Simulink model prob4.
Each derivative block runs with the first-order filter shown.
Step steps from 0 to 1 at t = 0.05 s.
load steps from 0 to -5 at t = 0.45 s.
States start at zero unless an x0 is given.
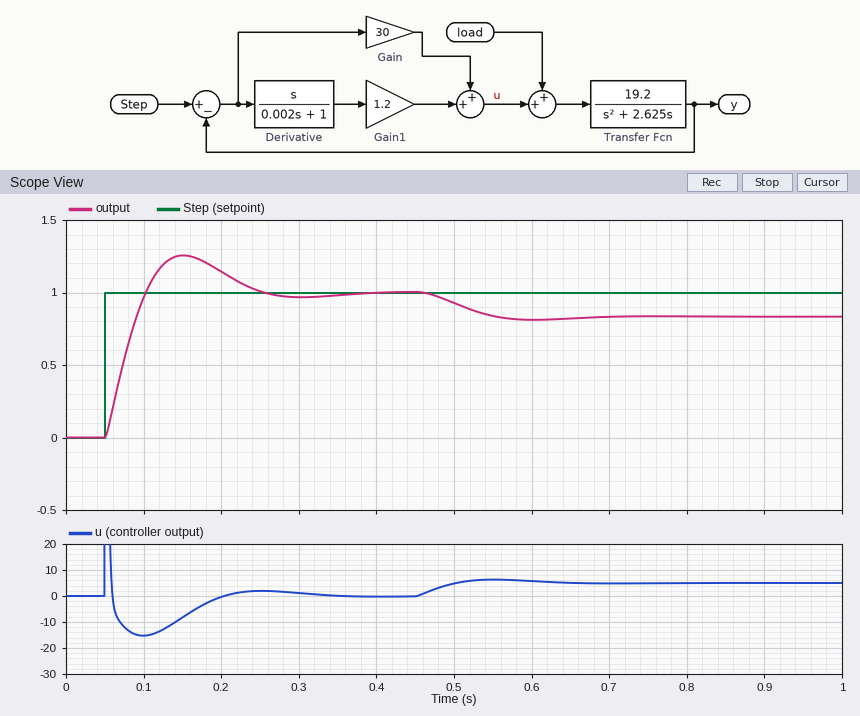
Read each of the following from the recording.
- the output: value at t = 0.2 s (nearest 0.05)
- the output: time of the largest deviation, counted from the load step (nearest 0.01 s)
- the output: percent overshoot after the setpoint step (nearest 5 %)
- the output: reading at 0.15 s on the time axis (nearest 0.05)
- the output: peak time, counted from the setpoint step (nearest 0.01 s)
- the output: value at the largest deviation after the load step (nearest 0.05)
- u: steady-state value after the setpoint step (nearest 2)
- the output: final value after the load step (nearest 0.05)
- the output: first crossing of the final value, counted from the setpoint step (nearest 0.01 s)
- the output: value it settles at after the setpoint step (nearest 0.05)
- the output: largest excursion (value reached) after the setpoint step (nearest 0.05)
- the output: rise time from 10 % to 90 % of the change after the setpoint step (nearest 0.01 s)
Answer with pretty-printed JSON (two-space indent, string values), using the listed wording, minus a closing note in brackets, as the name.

{
  "the output: value at t = 0.2 s": "1.15",
  "the output: time of the largest deviation, counted from the load step": "0.15 s",
  "the output: percent overshoot after the setpoint step": "25 %",
  "the output: reading at 0.15 s on the time axis": "1.25",
  "the output: peak time, counted from the setpoint step": "0.10 s",
  "the output: value at the largest deviation after the load step": "0.80",
  "u: steady-state value after the setpoint step": "0",
  "the output: final value after the load step": "0.85",
  "the output: first crossing of the final value, counted from the setpoint step": "0.05 s",
  "the output: value it settles at after the setpoint step": "1.00",
  "the output: largest excursion (value reached) after the setpoint step": "1.25",
  "the output: rise time from 10 % to 90 % of the change after the setpoint step": "0.04 s"
}
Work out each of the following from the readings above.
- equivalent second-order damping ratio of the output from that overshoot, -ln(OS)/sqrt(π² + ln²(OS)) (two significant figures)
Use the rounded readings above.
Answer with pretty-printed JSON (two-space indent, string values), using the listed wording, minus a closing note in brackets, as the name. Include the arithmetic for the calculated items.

{
  "equivalent second-order damping ratio of the output from that overshoot, -ln(OS)/sqrt(π² + ln²(OS))": "ln(0.25) = -1.386; 1.386 / sqrt(9.870 + 1.922) = 0.40"
}
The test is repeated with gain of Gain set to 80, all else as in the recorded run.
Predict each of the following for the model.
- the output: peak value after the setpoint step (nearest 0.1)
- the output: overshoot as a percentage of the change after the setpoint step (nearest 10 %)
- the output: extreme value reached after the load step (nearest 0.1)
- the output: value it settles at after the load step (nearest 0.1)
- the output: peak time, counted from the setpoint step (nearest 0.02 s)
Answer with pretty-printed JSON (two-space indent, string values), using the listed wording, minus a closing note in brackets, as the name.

{
  "the output: peak value after the setpoint step": "1.4",
  "the output: overshoot as a percentage of the change after the setpoint step": "40 %",
  "the output: extreme value reached after the load step": "0.9",
  "the output: value it settles at after the load step": "0.9",
  "the output: peak time, counted from the setpoint step": "0.06 s"
}
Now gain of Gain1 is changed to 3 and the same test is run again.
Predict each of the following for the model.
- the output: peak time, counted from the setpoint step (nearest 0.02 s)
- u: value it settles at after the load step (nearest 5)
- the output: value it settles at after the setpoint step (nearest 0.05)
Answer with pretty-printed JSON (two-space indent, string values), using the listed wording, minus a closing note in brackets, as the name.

{
  "the output: peak time, counted from the setpoint step": "0.08 s",
  "u: value it settles at after the load step": "5",
  "the output: value it settles at after the setpoint step": "1.00"
}
